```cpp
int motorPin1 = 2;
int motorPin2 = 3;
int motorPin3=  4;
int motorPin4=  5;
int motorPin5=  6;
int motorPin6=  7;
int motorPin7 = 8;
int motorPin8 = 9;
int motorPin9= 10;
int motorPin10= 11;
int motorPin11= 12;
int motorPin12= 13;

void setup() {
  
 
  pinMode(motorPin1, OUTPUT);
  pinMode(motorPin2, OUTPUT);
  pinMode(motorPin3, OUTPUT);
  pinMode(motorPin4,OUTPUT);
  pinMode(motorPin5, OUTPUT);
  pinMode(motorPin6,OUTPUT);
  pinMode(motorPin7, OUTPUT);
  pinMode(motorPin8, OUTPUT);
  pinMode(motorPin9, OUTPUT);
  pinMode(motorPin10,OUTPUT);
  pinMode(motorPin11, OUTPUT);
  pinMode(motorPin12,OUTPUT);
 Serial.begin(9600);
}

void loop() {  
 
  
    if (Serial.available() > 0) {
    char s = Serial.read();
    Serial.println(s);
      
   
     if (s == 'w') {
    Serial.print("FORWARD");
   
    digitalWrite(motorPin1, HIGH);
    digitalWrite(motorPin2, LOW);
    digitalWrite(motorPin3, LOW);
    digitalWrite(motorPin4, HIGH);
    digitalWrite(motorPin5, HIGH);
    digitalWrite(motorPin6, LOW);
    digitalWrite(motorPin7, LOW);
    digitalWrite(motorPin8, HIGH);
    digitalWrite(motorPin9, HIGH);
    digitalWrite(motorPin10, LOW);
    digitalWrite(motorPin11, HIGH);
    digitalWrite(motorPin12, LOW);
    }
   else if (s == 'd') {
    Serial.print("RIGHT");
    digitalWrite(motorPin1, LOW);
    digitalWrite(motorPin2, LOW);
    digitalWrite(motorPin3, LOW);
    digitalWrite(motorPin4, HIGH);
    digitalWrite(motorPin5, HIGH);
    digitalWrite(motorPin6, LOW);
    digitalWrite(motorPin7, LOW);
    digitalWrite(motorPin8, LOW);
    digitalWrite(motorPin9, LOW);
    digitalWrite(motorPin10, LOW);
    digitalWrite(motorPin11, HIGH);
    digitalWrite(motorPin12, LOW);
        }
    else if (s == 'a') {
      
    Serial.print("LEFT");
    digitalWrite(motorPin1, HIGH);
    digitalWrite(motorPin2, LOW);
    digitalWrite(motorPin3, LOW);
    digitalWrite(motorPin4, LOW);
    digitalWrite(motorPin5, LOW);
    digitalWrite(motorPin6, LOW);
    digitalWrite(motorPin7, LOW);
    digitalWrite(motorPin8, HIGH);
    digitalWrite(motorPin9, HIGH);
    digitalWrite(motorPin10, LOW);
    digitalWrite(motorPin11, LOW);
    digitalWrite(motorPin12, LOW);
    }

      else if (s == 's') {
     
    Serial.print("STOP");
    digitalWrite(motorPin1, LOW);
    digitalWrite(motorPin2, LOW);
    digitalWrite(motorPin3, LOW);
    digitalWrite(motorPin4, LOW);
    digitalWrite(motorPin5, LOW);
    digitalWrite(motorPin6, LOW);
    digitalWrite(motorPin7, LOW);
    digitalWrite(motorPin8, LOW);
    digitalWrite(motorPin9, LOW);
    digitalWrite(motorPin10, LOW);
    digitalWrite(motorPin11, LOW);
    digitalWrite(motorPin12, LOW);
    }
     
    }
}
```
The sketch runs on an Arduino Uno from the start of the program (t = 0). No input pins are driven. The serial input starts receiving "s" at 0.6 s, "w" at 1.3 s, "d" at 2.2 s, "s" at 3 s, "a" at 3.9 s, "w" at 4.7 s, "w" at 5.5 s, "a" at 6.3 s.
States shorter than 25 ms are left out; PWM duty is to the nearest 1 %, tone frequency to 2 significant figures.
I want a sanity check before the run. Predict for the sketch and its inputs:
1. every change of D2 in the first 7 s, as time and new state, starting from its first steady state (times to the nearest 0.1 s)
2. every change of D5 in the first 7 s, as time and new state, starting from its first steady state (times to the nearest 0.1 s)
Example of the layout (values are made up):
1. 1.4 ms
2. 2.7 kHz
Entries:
1. 0 s low; 1.3 s high; 2.2 s low; 3.9 s high
2. 0 s low; 1.3 s high; 3 s low; 4.7 s high; 6.3 s low
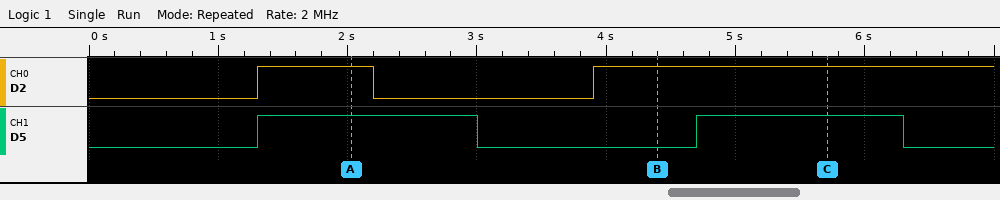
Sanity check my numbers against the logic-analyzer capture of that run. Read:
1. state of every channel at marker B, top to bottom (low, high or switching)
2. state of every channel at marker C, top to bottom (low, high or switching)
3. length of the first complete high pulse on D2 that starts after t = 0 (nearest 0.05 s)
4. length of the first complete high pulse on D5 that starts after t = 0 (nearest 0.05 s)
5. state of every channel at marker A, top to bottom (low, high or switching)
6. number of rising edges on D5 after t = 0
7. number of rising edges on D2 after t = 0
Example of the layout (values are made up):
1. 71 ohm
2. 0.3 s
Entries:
1. D2 high, D5 low
2. D2 high, D5 high
3. 0.90 s
4. 1.70 s
5. D2 high, D5 high
6. 2
7. 2
